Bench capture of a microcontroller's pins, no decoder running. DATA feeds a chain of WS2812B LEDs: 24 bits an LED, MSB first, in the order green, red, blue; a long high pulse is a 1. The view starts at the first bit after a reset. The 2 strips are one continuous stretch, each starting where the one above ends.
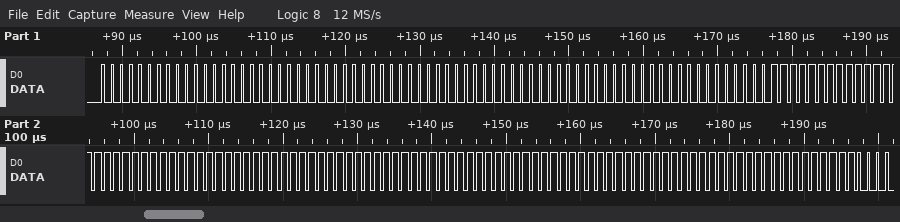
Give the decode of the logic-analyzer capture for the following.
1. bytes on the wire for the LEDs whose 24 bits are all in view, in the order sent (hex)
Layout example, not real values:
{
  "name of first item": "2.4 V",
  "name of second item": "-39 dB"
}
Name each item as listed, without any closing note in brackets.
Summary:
{
  "bytes on the wire for the LEDs whose 24 bits are all in view, in the order sent": "00 00 00 00 00 00 00 00 00 FF FF FF FF FF FF FF FF FF FF FF FF"
}
